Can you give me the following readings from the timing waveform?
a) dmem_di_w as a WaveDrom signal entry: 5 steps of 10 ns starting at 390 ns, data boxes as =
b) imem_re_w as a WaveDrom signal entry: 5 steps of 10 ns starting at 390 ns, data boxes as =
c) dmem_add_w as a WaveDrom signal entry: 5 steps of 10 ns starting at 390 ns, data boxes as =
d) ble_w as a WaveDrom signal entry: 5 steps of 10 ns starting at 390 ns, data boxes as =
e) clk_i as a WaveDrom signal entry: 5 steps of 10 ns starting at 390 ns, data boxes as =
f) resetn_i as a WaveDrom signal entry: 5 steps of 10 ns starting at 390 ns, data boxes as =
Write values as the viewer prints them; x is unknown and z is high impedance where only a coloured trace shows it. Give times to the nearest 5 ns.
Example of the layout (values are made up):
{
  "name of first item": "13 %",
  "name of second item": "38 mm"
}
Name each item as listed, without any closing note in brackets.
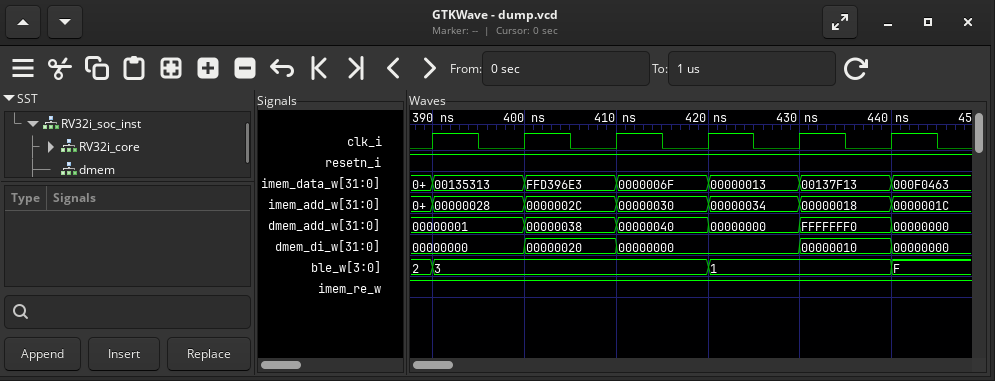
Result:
{
  "dmem_di_w as a WaveDrom signal entry: 5 steps of 10 ns starting at 390 ns, data boxes as =": "{name: 'dmem_di_w', wave: '===.=', data: '00000000 00000020 00000000 00000010'}",
  "imem_re_w as a WaveDrom signal entry: 5 steps of 10 ns starting at 390 ns, data boxes as =": "{name: 'imem_re_w', wave: '1....'}",
  "dmem_add_w as a WaveDrom signal entry: 5 steps of 10 ns starting at 390 ns, data boxes as =": "{name: 'dmem_add_w', wave: '=====', data: '00000001 00000038 00000040 00000000 FFFFFFF0'}",
  "ble_w as a WaveDrom signal entry: 5 steps of 10 ns starting at 390 ns, data boxes as =": "{name: 'ble_w', wave: '=..=.', data: '3 1'}",
  "clk_i as a WaveDrom signal entry: 5 steps of 10 ns starting at 390 ns, data boxes as =": "{name: 'clk_i', wave: 'p....'}",
  "resetn_i as a WaveDrom signal entry: 5 steps of 10 ns starting at 390 ns, data boxes as =": "{name: 'resetn_i', wave: '1....'}"
}
